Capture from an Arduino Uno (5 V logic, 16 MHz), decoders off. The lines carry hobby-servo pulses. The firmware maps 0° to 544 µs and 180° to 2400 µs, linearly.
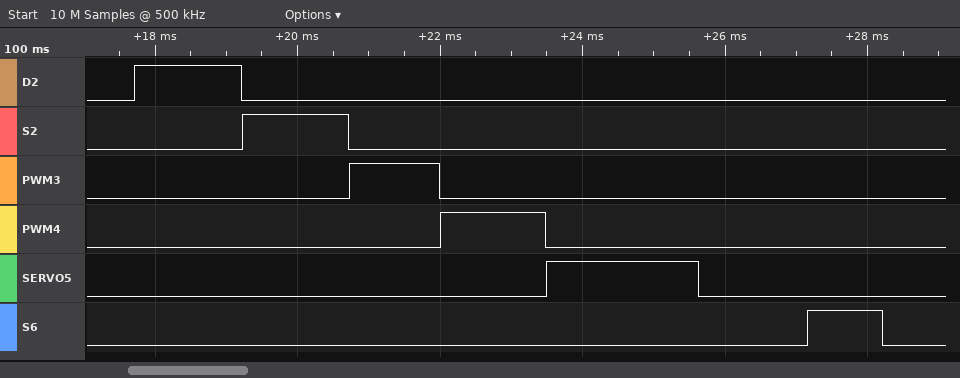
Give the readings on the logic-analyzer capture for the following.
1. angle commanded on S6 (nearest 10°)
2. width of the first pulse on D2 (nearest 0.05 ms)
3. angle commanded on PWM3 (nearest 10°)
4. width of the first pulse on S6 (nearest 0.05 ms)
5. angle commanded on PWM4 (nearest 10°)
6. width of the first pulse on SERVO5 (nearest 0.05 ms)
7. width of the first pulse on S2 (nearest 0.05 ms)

50°
1.50 ms
70°
1.05 ms
90°
2.15 ms
1.50 ms
